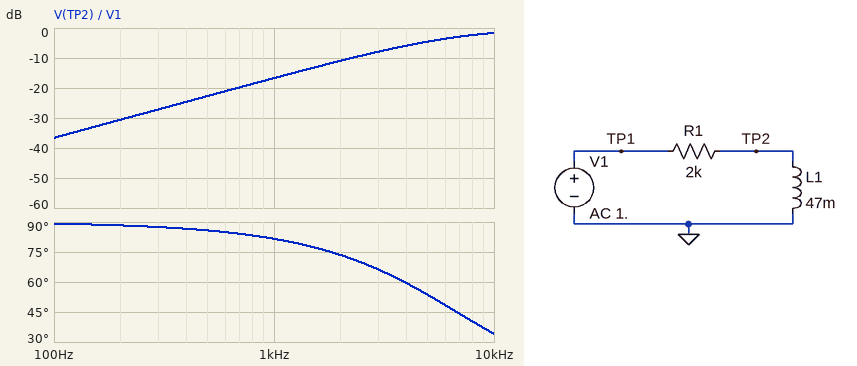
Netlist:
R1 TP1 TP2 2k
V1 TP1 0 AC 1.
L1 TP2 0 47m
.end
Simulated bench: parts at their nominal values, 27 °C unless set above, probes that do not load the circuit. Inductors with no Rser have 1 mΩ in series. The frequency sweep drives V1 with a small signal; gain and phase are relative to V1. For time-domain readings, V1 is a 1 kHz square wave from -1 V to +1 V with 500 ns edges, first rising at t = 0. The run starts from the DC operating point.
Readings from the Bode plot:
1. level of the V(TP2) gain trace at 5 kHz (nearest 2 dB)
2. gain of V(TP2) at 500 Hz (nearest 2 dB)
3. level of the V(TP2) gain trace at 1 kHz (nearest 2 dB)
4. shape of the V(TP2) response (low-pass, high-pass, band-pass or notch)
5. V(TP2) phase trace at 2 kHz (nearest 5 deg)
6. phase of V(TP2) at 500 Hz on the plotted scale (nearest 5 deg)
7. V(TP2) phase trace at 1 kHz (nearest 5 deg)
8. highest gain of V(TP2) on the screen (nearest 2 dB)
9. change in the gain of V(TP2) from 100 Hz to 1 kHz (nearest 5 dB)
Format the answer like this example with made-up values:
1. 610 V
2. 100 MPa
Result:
1. -4 dB
2. -22 dB
3. -16 dB
4. high-pass
5. 75 deg
6. 85 deg
7. 80 deg
8. -2 dB
9. 20 dB
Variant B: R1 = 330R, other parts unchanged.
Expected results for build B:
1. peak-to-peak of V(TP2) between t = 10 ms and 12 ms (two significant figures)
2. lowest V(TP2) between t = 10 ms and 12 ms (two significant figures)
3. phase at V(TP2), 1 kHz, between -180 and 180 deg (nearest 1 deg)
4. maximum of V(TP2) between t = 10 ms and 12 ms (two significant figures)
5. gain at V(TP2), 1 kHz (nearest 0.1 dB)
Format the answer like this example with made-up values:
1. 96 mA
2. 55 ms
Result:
1. 3.9 V
2. -1.9 V
3. 48 deg
4. 1.9 V
5. -3.5 dB
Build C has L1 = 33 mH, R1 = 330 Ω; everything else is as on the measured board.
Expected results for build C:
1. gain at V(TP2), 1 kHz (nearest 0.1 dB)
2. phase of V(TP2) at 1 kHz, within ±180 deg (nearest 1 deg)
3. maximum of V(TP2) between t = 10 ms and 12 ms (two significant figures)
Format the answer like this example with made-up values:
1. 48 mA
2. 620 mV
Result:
1. -5.5 dB
2. 58 deg
3. 2.0 V
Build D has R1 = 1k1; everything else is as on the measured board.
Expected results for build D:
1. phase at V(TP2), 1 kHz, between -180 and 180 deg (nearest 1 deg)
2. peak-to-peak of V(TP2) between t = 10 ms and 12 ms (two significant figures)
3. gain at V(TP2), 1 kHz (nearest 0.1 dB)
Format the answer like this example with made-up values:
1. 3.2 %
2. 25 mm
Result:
1. 75 deg
2. 4.0 V
3. -11.7 dB
